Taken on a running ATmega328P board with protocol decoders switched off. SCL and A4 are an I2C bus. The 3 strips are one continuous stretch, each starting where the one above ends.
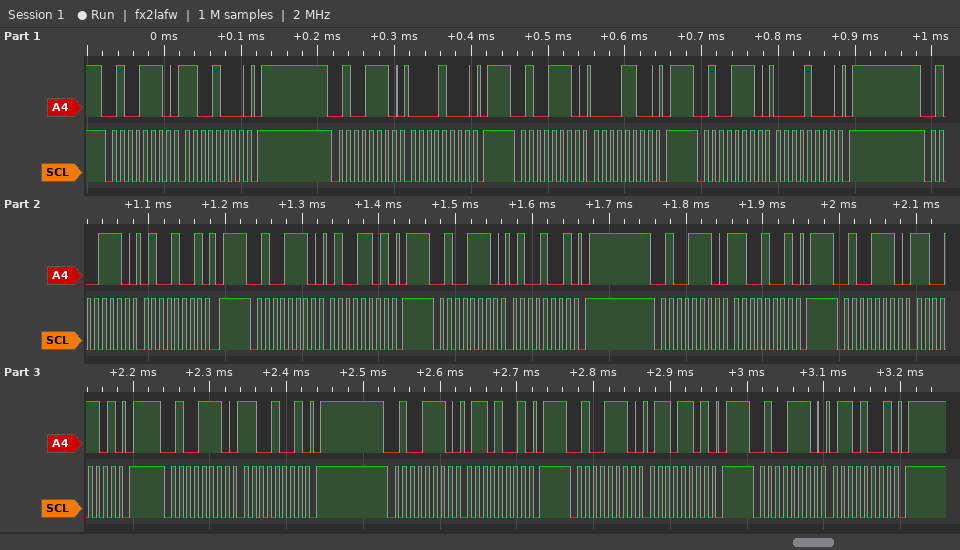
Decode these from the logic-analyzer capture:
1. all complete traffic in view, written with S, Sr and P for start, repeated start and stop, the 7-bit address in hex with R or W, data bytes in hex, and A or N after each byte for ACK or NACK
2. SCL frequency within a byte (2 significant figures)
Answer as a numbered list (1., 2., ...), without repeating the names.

1. S 27W A C8 A P S 27W A 08 A P S 27W A 0C A P S 27W A 08 A P S 27W A 49 A P S 27W A 4D A P S 27W A 49 A P S 27W A C9 A P S 27W A CD A P S 27W A C9 A P S 27W A 69 A P S 27W A 6D A P S 27W A 69 A P
2. 100 kHz
